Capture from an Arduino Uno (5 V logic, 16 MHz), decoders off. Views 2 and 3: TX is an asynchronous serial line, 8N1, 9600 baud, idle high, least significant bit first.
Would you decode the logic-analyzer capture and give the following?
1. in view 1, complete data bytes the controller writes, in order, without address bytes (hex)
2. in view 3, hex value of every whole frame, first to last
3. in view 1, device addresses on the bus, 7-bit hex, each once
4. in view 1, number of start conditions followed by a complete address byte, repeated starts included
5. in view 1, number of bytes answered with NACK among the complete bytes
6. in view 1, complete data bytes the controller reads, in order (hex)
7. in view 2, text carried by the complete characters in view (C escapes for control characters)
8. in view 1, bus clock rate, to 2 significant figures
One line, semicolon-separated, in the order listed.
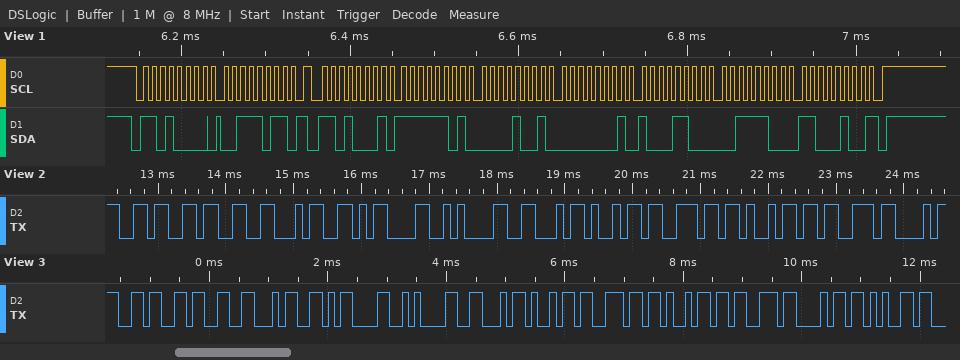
3B; 36 33 34 0D 0A 46 69 6E 69 73 68 65; 0x68; 2; 1; FD 09 01 8C 3C C4; "634\r\nFinis"; 100 kHz
